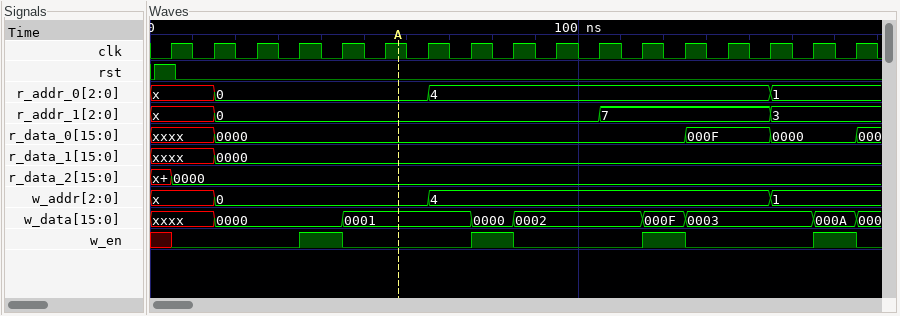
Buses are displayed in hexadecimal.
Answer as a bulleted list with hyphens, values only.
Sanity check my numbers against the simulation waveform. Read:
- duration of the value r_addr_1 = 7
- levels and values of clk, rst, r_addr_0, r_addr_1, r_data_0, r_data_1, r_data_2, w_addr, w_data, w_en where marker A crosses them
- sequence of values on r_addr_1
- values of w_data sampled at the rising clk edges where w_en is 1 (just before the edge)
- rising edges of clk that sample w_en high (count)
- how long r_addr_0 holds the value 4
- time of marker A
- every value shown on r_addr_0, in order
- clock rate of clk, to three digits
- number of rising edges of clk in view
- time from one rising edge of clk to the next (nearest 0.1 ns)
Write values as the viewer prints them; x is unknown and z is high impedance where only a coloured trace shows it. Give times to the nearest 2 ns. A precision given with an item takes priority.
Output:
- 40 ns
- clk=1, rst=0, r_addr_0=0, r_addr_1=0, r_data_0=0000, r_data_1=0000, r_data_2=0000, w_addr=0, w_data=0001, w_en=0
- x, 0, 7, 3
- 0000, 0000, 000F, 000A
- 4
- 80 ns
- 58 ns
- x, 0, 4, 1
- 100 MHz
- 17
- 10 ns
